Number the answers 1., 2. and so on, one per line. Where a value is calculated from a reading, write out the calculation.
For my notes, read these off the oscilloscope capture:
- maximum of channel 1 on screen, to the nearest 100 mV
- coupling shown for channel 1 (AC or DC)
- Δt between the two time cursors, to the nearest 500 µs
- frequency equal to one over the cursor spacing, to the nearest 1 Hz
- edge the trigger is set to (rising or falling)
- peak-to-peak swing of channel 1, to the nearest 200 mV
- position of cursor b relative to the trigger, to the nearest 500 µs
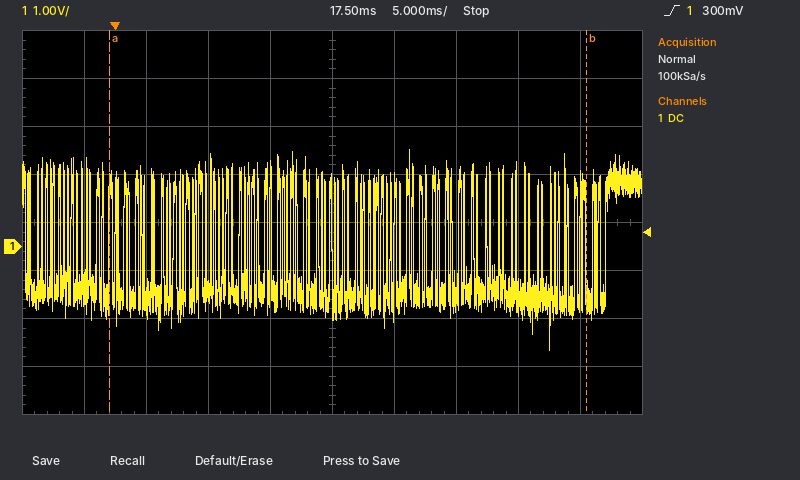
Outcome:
1. 2.0 V
2. DC
3. 38.5 ms
4. 1 / 38.5 ms ≈ 26 Hz
5. rising
6. 4.2 V
7. +38.0 ms
